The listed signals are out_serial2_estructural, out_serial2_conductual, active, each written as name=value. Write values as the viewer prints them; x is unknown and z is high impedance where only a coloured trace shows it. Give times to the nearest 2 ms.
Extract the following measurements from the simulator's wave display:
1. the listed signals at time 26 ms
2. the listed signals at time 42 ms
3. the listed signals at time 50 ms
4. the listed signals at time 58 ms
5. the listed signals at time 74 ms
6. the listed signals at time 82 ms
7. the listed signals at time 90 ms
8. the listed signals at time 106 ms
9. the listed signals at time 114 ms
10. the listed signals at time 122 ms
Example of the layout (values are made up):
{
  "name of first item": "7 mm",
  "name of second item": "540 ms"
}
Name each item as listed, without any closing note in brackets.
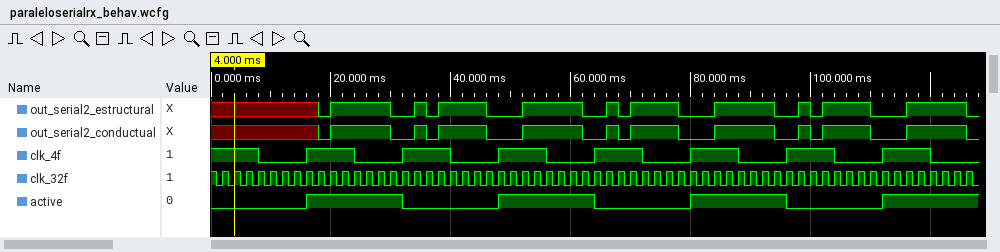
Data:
{
  "the listed signals at time 26 ms": "out_serial2_estructural=1, out_serial2_conductual=1, active=1",
  "the listed signals at time 42 ms": "out_serial2_estructural=1, out_serial2_conductual=1, active=0",
  "the listed signals at time 50 ms": "out_serial2_estructural=0, out_serial2_conductual=0, active=1",
  "the listed signals at time 58 ms": "out_serial2_estructural=1, out_serial2_conductual=1, active=1",
  "the listed signals at time 74 ms": "out_serial2_estructural=1, out_serial2_conductual=1, active=0",
  "the listed signals at time 82 ms": "out_serial2_estructural=0, out_serial2_conductual=0, active=1",
  "the listed signals at time 90 ms": "out_serial2_estructural=1, out_serial2_conductual=1, active=1",
  "the listed signals at time 106 ms": "out_serial2_estructural=1, out_serial2_conductual=1, active=0",
  "the listed signals at time 114 ms": "out_serial2_estructural=0, out_serial2_conductual=0, active=1",
  "the listed signals at time 122 ms": "out_serial2_estructural=1, out_serial2_conductual=1, active=1"
}
